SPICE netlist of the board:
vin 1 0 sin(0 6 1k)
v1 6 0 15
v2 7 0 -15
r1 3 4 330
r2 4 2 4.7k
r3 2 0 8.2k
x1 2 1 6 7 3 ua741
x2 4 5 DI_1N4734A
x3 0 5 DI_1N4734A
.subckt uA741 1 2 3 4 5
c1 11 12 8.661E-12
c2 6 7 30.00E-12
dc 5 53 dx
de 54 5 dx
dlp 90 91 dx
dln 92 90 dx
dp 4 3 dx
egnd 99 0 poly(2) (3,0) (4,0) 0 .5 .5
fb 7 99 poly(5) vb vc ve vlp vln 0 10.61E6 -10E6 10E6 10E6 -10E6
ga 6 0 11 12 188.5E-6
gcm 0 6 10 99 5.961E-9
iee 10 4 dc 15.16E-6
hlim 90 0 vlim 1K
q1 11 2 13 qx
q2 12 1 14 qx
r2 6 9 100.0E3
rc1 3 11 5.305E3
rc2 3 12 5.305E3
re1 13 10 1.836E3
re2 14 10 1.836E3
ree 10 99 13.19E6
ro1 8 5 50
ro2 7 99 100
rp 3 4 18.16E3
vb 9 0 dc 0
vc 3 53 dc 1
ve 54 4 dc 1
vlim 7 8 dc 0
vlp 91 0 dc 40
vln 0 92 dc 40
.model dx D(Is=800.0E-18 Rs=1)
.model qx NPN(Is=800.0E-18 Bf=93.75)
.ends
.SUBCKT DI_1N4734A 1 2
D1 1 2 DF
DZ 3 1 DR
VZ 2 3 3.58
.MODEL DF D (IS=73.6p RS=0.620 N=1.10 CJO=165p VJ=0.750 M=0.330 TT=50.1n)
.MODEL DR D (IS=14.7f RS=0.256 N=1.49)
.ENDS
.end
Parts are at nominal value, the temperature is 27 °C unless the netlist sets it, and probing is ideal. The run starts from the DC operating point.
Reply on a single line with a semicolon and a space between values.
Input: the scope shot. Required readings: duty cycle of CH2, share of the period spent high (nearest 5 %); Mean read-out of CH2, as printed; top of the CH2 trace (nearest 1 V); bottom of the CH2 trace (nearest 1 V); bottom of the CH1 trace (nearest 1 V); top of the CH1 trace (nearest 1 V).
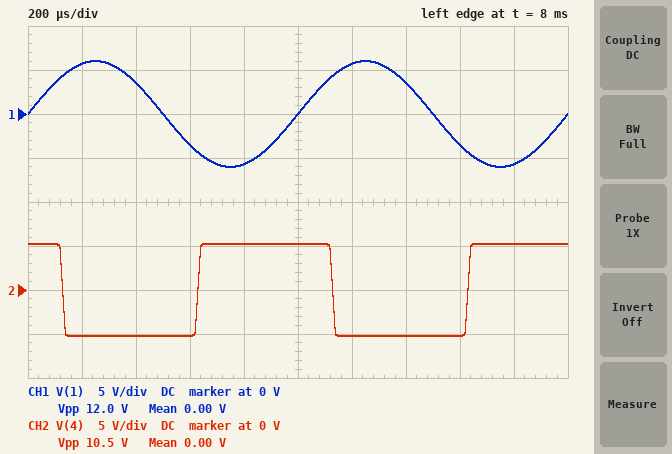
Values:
50 %; 0.00 V; 5 V; -5 V; -6 V; 6 V
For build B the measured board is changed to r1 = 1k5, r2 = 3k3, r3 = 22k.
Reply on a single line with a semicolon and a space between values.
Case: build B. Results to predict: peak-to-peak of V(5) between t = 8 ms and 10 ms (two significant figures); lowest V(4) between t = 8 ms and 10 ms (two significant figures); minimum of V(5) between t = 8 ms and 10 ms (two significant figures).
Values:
5.1 V; -5.1 V; -520 mV
